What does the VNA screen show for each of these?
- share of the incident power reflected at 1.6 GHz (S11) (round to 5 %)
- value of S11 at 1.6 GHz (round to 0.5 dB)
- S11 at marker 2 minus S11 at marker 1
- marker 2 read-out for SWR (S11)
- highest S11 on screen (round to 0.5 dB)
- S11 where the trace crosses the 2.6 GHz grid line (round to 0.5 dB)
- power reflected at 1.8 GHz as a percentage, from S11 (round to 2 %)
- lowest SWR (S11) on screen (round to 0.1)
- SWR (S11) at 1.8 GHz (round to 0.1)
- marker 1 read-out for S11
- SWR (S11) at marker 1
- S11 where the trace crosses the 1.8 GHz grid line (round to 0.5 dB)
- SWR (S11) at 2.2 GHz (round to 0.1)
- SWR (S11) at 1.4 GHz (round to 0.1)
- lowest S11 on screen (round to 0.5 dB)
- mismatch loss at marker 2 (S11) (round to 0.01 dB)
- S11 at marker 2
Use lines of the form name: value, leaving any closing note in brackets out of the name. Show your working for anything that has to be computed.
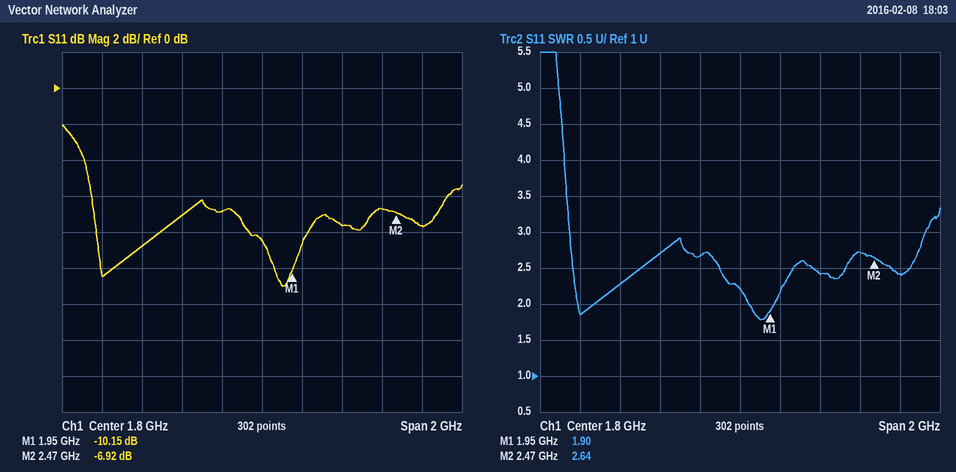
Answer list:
share of the incident power reflected at 1.6 GHz (S11): 10^(-7/10) ≈ 20 %
value of S11 at 1.6 GHz: -7.0 dB
S11 at marker 2 minus S11 at marker 1: -6.92 − (-10.15) = 3.23 dB
marker 2 read-out for SWR: 2.64
highest S11 on screen: -2.0 dB
S11 where the trace crosses the 2.6 GHz grid line: -7.5 dB
power reflected at 1.8 GHz as a percentage, from S11: 10^(-8.5/10) ≈ 14 %
lowest SWR (S11) on screen: 1.8
SWR (S11) at 1.8 GHz: 2.2
marker 1 read-out for S11: -10.15 dB
SWR (S11) at marker 1: 1.90
S11 where the trace crosses the 1.8 GHz grid line: -8.5 dB
SWR (S11) at 2.2 GHz: 2.4
SWR (S11) at 1.4 GHz: 2.7
lowest S11 on screen: -11.0 dB
mismatch loss at marker 2 (S11): −10 log10(1 − 10^(-6.92/10)) ≈ 0.99 dB
S11 at marker 2: -6.92 dB
